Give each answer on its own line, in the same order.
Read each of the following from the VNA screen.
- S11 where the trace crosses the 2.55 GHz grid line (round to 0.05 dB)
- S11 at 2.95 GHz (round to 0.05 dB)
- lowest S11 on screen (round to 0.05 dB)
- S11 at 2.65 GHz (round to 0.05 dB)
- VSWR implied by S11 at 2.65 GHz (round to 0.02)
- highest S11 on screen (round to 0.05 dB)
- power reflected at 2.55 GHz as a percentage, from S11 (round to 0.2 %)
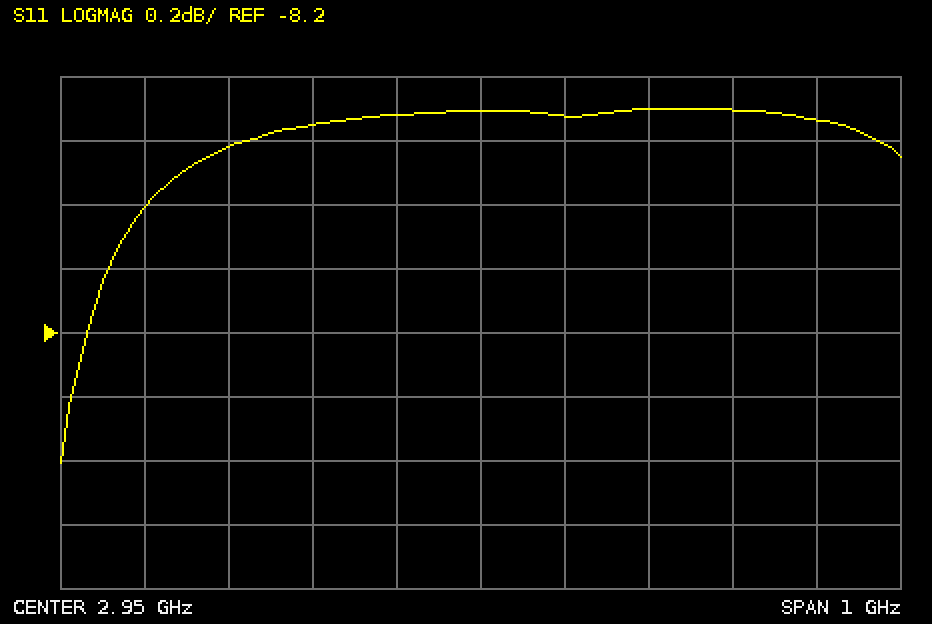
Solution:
-7.80 dB
-7.50 dB
-8.60 dB
-7.60 dB
2.42
-7.50 dB
16.6 %
